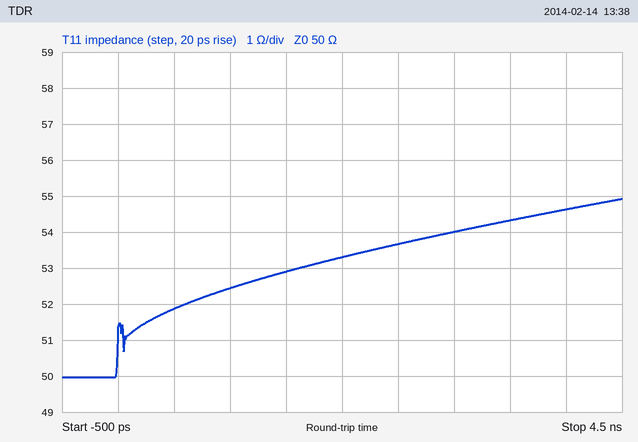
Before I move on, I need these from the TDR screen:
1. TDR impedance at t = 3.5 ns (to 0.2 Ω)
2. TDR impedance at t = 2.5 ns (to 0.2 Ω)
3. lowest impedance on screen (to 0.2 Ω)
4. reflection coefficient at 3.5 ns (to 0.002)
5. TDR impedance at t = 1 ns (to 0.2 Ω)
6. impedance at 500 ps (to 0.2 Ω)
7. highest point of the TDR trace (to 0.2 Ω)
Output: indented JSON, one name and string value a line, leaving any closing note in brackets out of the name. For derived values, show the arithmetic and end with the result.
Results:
{
  "TDR impedance at t = 3.5 ns": "54.4 Ω",
  "TDR impedance at t = 2.5 ns": "53.6 Ω",
  "lowest impedance on screen": "50.0 Ω",
  "reflection coefficient at 3.5 ns": "(54.4 − 50)/(54.4 + 50) ≈ +0.042",
  "TDR impedance at t = 1 ns": "52.4 Ω",
  "impedance at 500 ps": "51.8 Ω",
  "highest point of the TDR trace": "55.0 Ω"
}
